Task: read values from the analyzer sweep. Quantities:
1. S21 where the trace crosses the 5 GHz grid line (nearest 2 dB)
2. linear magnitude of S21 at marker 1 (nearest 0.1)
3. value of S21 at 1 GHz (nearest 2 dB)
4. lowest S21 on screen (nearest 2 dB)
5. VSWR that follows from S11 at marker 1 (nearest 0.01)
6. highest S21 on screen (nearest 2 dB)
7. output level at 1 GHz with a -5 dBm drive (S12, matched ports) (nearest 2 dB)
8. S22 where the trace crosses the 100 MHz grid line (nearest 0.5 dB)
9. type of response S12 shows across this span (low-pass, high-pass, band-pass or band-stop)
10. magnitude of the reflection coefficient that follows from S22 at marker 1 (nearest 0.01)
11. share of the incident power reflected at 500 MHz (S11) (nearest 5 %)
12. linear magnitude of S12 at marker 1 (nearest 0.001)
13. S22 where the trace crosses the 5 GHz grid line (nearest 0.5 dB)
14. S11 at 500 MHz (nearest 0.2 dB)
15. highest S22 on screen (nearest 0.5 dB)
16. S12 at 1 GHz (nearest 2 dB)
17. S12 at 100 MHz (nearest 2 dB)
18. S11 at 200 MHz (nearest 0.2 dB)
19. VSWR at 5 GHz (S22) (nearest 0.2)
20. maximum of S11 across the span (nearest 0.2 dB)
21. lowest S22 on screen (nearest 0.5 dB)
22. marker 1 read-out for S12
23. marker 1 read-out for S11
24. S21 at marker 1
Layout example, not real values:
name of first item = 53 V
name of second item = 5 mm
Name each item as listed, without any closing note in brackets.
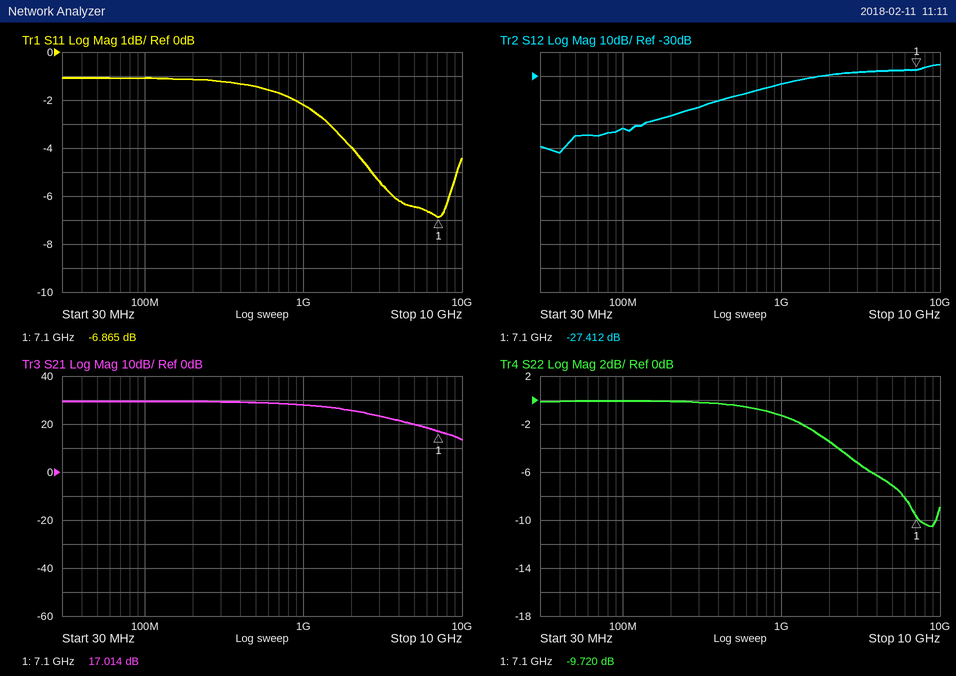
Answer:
S21 where the trace crosses the 5 GHz grid line = 20 dB
linear magnitude of S21 at marker 1 = 7.1
value of S21 at 1 GHz = 28 dB
lowest S21 on screen = 14 dB
VSWR that follows from S11 at marker 1 = 2.66
highest S21 on screen = 30 dB
output level at 1 GHz with a -5 dBm drive (S12, matched ports) = -38 dBm
S22 where the trace crosses the 100 MHz grid line = 0.0 dB
type of response S12 shows across this span = high-pass
magnitude of the reflection coefficient that follows from S22 at marker 1 = 0.33
share of the incident power reflected at 500 MHz (S11) = 70 %
linear magnitude of S12 at marker 1 = 0.043
S22 where the trace crosses the 5 GHz grid line = -7.0 dB
S11 at 500 MHz = -1.4 dB
highest S22 on screen = 0.0 dB
S12 at 1 GHz = -34 dB
S12 at 100 MHz = -52 dB
S11 at 200 MHz = -1.2 dB
VSWR at 5 GHz (S22) = 2.6
maximum of S11 across the span = -1.0 dB
lowest S22 on screen = -10.5 dB
marker 1 read-out for S12 = -27.412 dB
marker 1 read-out for S11 = -6.865 dB
S21 at marker 1 = 17.014 dB
